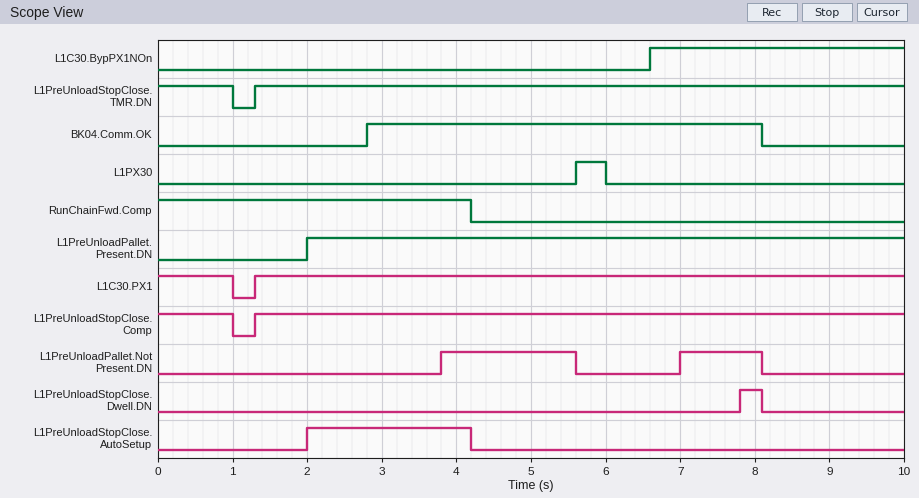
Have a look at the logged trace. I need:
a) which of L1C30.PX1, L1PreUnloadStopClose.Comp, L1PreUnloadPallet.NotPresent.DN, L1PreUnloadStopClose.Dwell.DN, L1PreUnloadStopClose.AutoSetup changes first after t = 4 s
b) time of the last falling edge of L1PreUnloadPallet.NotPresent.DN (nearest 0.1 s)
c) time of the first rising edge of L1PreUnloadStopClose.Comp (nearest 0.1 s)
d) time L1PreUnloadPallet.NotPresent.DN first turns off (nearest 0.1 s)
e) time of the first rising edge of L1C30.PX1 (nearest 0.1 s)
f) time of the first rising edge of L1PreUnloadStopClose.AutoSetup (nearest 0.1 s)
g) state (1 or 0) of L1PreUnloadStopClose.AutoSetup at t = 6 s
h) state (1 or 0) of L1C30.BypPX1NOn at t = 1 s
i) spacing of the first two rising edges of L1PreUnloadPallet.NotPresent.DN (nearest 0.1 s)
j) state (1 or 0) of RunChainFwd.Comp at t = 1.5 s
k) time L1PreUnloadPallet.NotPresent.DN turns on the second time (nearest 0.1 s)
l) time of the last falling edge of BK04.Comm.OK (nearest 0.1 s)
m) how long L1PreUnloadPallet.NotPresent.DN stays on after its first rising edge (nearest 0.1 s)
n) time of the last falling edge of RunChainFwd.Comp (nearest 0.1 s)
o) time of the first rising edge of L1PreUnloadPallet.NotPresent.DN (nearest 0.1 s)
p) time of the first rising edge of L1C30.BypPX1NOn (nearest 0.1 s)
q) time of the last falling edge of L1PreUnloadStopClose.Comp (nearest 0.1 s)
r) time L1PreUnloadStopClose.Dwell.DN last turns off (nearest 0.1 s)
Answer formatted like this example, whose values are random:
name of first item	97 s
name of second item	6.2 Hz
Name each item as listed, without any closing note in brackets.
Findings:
which of L1C30.PX1, L1PreUnloadStopClose.Comp, L1PreUnloadPallet.NotPresent.DN, L1PreUnloadStopClose.Dwell.DN, L1PreUnloadStopClose.AutoSetup changes first after t = 4 s	L1PreUnloadStopClose.AutoSetup
time of the last falling edge of L1PreUnloadPallet.NotPresent.DN	8.1 s
time of the first rising edge of L1PreUnloadStopClose.Comp	1.3 s
time L1PreUnloadPallet.NotPresent.DN first turns off	5.6 s
time of the first rising edge of L1C30.PX1	1.3 s
time of the first rising edge of L1PreUnloadStopClose.AutoSetup	2.0 s
state (1 or 0) of L1PreUnloadStopClose.AutoSetup at t = 6 s	0
state (1 or 0) of L1C30.BypPX1NOn at t = 1 s	0
spacing of the first two rising edges of L1PreUnloadPallet.NotPresent.DN	3.2 s
state (1 or 0) of RunChainFwd.Comp at t = 1.5 s	1
time L1PreUnloadPallet.NotPresent.DN turns on the second time	7.0 s
time of the last falling edge of BK04.Comm.OK	8.1 s
how long L1PreUnloadPallet.NotPresent.DN stays on after its first rising edge	1.8 s
time of the last falling edge of RunChainFwd.Comp	4.2 s
time of the first rising edge of L1PreUnloadPallet.NotPresent.DN	3.8 s
time of the first rising edge of L1C30.BypPX1NOn	6.6 s
time of the last falling edge of L1PreUnloadStopClose.Comp	1.0 s
time L1PreUnloadStopClose.Dwell.DN last turns off	8.1 s
